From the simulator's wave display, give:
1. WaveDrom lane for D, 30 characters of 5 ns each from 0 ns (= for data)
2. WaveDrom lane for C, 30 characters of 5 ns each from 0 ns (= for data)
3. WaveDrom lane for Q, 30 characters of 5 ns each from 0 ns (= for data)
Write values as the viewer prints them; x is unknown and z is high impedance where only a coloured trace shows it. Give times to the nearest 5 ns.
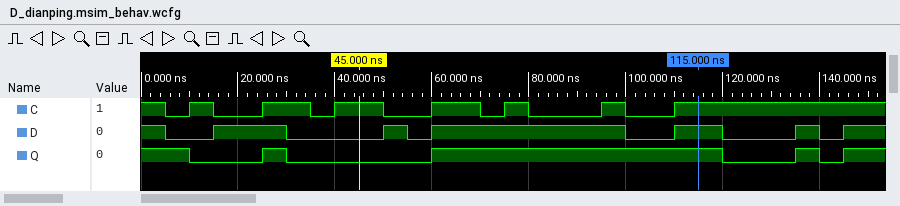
{name: 'D', wave: '10.1..0...101.......0.1.0..101'}
{name: 'C', wave: '1010.1.01.0.1.010..10.1.......'}
{name: 'Q', wave: '1.0..10.....1...........0..101'}
